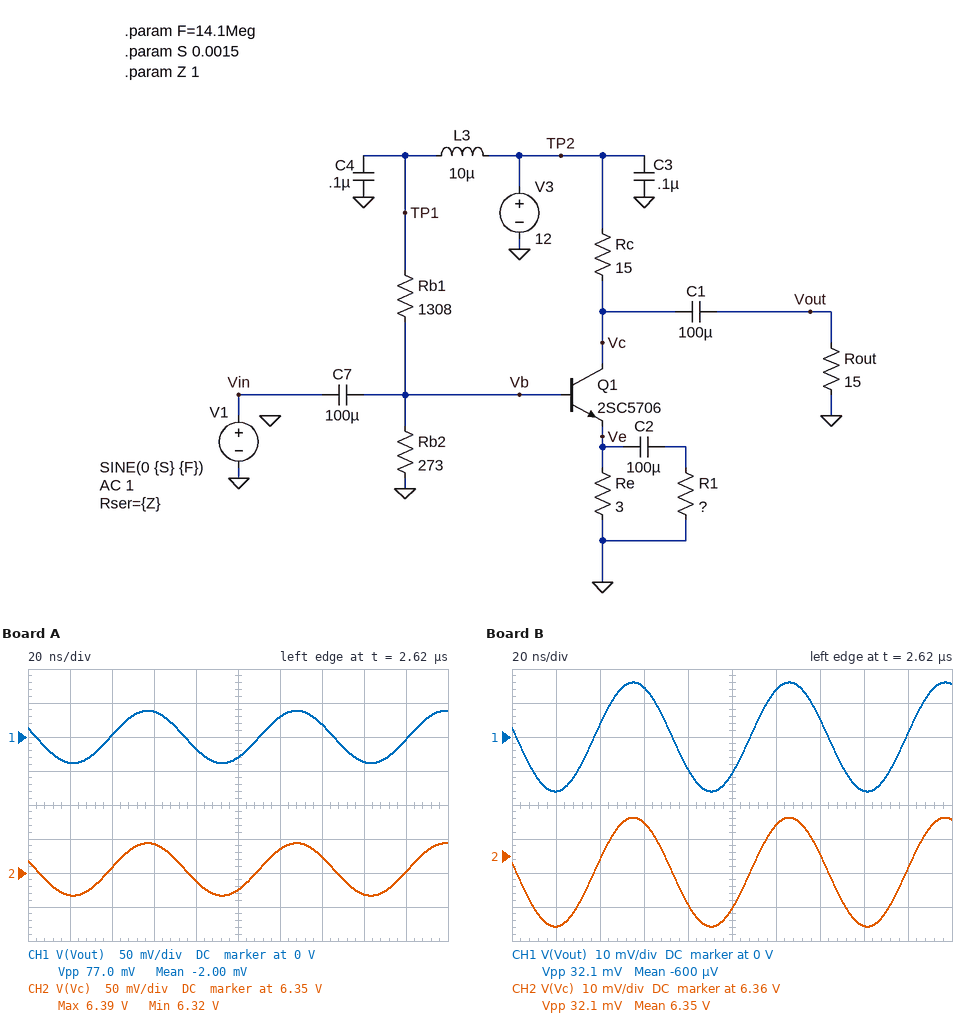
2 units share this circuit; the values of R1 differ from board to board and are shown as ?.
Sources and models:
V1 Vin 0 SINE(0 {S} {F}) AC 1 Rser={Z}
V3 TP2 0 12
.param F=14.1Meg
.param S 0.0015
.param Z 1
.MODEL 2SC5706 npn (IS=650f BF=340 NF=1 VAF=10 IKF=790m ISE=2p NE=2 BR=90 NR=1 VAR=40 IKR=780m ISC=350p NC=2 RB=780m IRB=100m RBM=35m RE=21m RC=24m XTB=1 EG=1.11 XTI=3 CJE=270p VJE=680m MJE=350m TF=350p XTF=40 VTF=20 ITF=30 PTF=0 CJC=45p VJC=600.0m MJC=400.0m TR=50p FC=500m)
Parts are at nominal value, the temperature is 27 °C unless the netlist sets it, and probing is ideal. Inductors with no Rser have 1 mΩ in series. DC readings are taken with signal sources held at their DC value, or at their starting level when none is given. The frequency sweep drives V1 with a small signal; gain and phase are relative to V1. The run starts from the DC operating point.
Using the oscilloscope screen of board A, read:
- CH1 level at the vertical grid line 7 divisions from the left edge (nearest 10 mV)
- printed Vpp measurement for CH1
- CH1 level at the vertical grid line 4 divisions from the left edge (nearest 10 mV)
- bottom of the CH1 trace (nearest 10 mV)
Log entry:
20 mV
77.0 mV
-20 mV
-40 mV
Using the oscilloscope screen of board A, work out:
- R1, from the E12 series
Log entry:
0.15 Ω
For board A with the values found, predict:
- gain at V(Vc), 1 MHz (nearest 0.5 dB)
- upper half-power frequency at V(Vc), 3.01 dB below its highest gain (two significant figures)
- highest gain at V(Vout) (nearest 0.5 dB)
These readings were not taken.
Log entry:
28.5 dB
42 MHz
28.5 dB
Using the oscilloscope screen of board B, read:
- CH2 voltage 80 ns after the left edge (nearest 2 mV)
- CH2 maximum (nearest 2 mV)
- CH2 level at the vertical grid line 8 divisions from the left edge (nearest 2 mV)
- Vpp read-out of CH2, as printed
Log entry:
6.346 V
6.372 V
6.340 V
32.1 mV
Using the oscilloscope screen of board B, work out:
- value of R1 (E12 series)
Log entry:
0.68 Ω
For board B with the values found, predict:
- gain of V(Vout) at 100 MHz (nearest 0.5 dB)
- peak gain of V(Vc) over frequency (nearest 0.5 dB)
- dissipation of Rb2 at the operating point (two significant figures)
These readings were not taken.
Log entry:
17.0 dB
20.5 dB
12 mW
